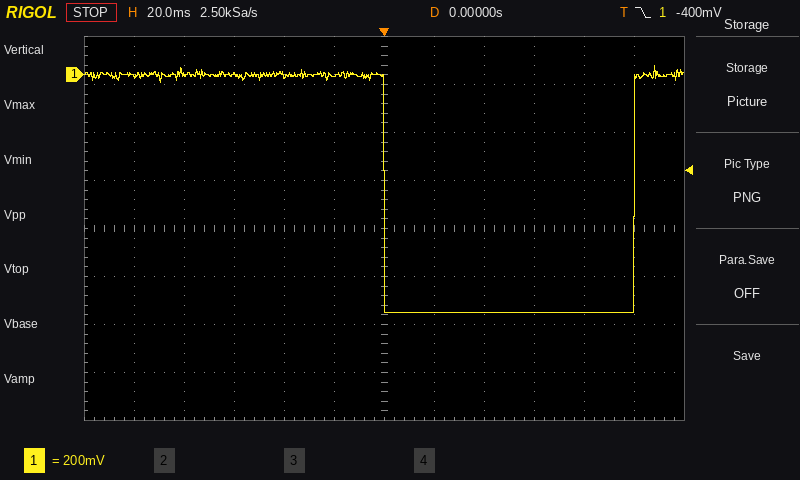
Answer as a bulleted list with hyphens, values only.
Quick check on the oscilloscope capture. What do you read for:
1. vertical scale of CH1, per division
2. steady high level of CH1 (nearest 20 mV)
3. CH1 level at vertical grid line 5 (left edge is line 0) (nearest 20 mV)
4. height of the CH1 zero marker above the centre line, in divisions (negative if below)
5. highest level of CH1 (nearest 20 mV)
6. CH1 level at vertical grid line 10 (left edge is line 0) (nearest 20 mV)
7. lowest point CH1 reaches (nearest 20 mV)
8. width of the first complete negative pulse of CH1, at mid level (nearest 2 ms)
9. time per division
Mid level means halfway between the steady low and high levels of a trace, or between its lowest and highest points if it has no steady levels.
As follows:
- 200 mV
- 0 mV
- 0 mV
- +3.2 div
- 40 mV
- -1.00 V
- -1.00 V
- 100 ms
- 20 ms
